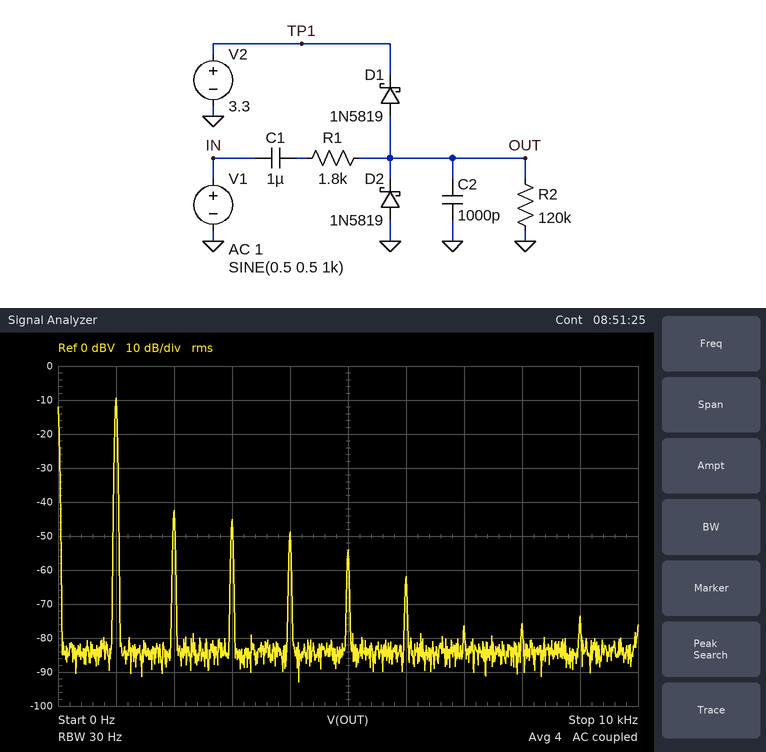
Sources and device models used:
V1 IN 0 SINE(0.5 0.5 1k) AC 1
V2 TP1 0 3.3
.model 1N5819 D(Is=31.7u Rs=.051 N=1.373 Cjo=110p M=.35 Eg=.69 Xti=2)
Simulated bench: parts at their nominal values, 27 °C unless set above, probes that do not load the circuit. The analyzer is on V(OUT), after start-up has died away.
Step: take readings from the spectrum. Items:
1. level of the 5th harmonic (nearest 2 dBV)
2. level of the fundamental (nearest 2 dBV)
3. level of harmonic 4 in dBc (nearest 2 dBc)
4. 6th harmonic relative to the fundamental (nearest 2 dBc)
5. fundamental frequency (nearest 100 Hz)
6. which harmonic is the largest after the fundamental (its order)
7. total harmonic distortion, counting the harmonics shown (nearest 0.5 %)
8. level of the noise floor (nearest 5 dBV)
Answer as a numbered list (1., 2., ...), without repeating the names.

1. -54 dBV
2. -10 dBV
3. -40 dBc
4. -52 dBc
5. 1.0 kHz
6. 2
7. 3.0 %
8. -85 dBV
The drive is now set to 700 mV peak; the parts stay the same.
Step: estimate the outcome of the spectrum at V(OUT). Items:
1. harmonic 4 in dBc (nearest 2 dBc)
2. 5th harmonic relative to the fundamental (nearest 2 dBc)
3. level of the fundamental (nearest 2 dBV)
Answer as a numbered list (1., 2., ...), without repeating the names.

1. -38 dBc
2. -42 dBc
3. -6 dBV
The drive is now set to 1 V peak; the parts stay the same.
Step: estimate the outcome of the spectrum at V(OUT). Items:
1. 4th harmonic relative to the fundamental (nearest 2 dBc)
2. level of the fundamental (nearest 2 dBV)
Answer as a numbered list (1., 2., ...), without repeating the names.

1. -38 dBc
2. -4 dBV
